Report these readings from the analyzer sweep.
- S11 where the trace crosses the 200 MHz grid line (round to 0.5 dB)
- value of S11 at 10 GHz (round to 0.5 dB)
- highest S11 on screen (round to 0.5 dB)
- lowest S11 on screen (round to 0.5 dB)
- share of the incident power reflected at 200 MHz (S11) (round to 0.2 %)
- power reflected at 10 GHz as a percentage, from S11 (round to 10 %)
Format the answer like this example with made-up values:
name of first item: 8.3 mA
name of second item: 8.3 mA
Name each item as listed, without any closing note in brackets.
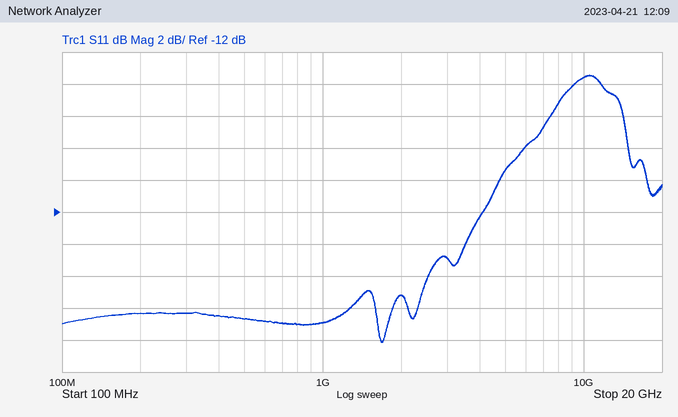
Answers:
S11 where the trace crosses the 200 MHz grid line: -18.5 dB
value of S11 at 10 GHz: -3.5 dB
highest S11 on screen: -3.5 dB
lowest S11 on screen: -20.0 dB
share of the incident power reflected at 200 MHz (S11): 1.4 %
power reflected at 10 GHz as a percentage, from S11: 40 %
